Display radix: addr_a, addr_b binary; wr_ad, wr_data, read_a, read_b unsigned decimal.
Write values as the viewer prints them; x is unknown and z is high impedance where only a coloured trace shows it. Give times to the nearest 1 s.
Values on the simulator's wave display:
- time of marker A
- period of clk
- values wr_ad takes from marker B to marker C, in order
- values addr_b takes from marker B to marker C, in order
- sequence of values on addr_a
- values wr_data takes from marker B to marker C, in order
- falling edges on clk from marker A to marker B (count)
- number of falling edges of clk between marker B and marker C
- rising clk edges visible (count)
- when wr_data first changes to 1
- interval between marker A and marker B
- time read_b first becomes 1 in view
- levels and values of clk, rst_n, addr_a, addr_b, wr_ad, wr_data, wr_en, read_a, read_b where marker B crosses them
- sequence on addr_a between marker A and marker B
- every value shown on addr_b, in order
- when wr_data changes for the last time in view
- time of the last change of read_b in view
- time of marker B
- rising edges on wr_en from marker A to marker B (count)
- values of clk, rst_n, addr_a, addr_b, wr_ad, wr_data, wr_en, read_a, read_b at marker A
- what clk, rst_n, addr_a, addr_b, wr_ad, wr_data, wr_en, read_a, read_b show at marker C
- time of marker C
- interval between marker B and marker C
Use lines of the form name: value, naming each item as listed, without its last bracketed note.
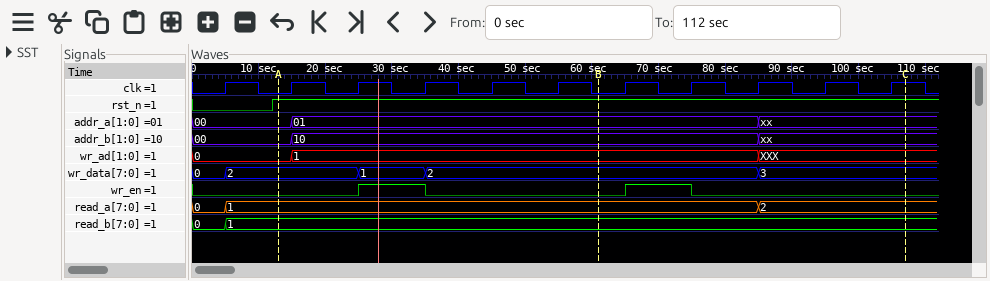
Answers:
time of marker A: 13 s
period of clk: 10 s
values wr_ad takes from marker B to marker C, in order: 1, XXX
values addr_b takes from marker B to marker C, in order: 10, xx
sequence of values on addr_a: 00, 01, xx
values wr_data takes from marker B to marker C, in order: 2, 3
falling edges on clk from marker A to marker B: 5
number of falling edges of clk between marker B and marker C: 4
rising clk edges visible: 11
when wr_data first changes to 1: 25 s
interval between marker A and marker B: 48 s
time read_b first becomes 1 in view: 5 s
levels and values of clk, rst_n, addr_a, addr_b, wr_ad, wr_data, wr_en, read_a, read_b where marker B crosses them: clk=0, rst_n=1, addr_a=01, addr_b=10, wr_ad=1, wr_data=2, wr_en=0, read_a=1, read_b=1
sequence on addr_a between marker A and marker B: 00, 01
every value shown on addr_b, in order: 00, 10, xx
when wr_data changes for the last time in view: 85 s
time of the last change of read_b in view: 5 s
time of marker B: 61 s
rising edges on wr_en from marker A to marker B: 1
values of clk, rst_n, addr_a, addr_b, wr_ad, wr_data, wr_en, read_a, read_b at marker A: clk=0, rst_n=1, addr_a=00, addr_b=00, wr_ad=0, wr_data=2, wr_en=0, read_a=1, read_b=1
what clk, rst_n, addr_a, addr_b, wr_ad, wr_data, wr_en, read_a, read_b show at marker C: clk=1, rst_n=1, addr_a=xx, addr_b=xx, wr_ad=XXX, wr_data=3, wr_en=0, read_a=2, read_b=1
time of marker C: 107 s
interval between marker B and marker C: 46 s
